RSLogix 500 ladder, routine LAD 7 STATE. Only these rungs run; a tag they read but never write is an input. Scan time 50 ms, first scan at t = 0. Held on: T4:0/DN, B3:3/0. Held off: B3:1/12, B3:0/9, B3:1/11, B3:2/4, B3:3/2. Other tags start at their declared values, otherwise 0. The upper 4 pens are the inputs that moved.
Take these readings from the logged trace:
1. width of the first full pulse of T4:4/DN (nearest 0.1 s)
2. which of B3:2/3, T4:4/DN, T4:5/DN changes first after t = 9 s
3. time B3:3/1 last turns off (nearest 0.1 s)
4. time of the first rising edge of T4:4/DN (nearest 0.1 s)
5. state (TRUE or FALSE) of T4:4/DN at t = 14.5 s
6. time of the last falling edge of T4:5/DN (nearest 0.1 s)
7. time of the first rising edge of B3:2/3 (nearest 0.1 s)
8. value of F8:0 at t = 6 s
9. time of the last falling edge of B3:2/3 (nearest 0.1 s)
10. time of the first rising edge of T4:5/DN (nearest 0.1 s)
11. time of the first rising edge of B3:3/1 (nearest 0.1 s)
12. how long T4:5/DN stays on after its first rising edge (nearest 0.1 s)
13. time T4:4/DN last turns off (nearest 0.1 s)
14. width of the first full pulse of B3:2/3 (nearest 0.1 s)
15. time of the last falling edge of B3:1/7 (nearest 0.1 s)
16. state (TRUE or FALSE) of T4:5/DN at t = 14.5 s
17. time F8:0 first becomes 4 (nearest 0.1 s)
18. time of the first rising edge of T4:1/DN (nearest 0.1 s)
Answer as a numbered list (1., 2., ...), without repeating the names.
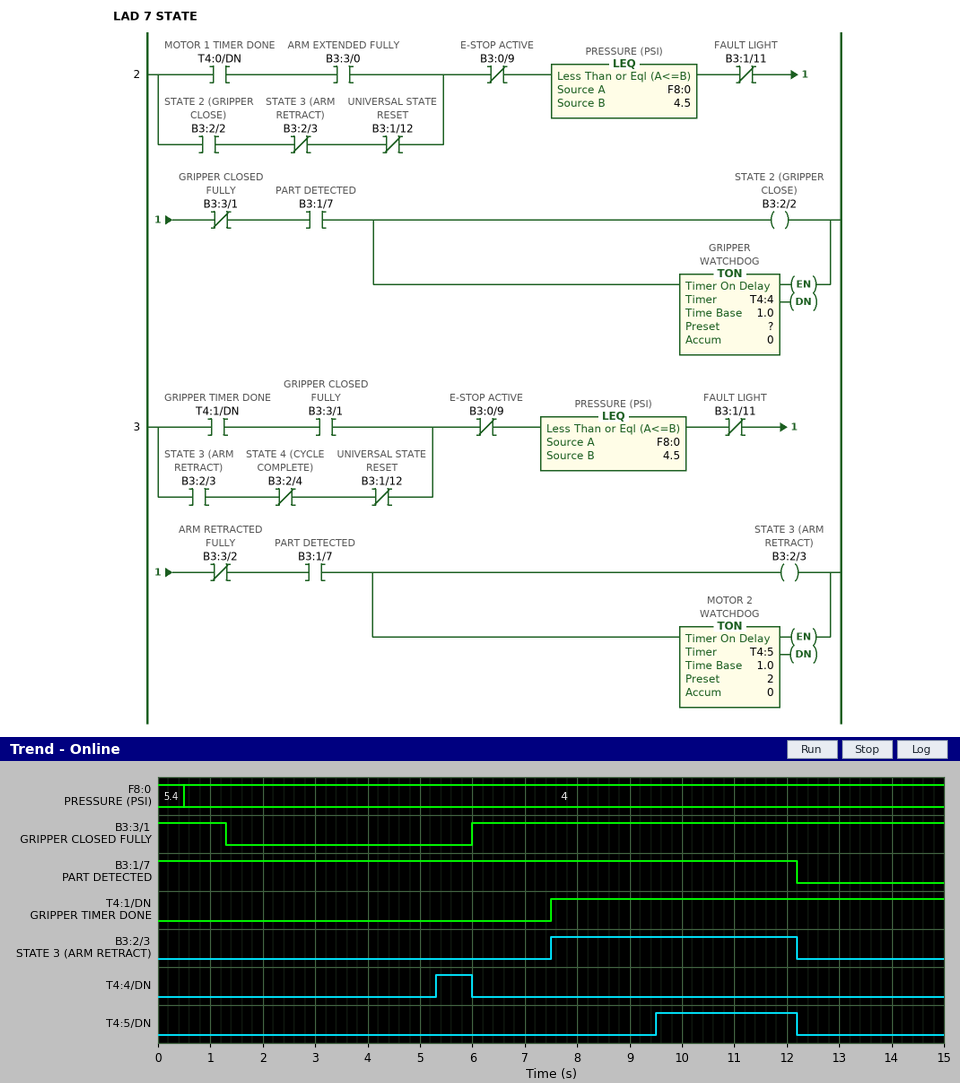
1. 0.7 s
2. T4:5/DN
3. 1.3 s
4. 5.3 s
5. FALSE
6. 12.2 s
7. 7.5 s
8. 4
9. 12.2 s
10. 9.5 s
11. 6.0 s
12. 2.7 s
13. 6.0 s
14. 4.7 s
15. 12.2 s
16. FALSE
17. 0.5 s
18. 7.5 s
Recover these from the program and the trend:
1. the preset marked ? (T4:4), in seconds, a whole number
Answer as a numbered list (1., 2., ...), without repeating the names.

1. 4 s
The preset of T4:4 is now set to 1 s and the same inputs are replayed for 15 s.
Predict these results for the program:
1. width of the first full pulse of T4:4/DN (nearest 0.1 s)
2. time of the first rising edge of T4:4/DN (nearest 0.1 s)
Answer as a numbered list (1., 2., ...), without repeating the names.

1. 3.7 s
2. 2.3 s
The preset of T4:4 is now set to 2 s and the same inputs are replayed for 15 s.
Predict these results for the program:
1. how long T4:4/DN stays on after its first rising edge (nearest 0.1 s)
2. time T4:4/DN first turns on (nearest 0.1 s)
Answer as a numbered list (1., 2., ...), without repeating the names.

1. 2.7 s
2. 3.3 s
